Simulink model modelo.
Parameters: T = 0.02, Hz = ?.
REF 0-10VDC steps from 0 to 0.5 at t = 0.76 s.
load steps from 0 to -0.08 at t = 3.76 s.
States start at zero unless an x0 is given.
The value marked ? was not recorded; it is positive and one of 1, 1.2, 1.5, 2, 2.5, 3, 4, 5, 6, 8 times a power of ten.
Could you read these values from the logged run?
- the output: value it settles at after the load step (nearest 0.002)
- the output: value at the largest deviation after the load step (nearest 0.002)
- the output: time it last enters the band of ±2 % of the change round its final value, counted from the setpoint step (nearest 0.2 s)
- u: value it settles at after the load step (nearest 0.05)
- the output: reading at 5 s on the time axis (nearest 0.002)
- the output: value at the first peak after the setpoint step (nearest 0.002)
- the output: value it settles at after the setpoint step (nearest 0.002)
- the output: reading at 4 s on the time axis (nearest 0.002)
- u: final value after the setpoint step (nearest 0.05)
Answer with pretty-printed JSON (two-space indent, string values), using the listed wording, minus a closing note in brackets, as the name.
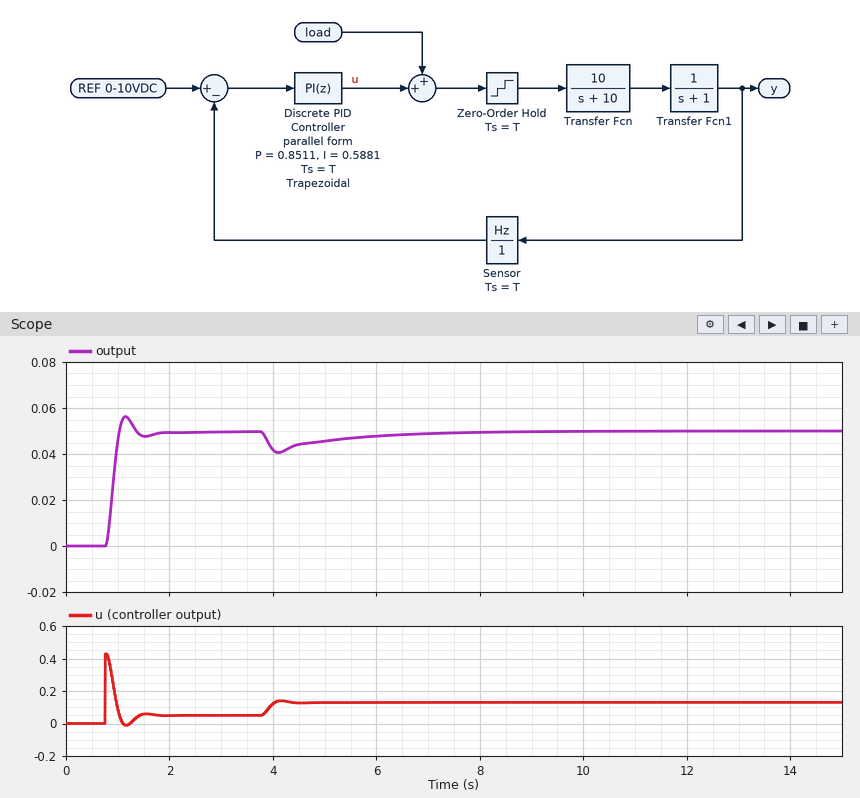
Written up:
{
  "the output: value it settles at after the load step": "0.050",
  "the output: value at the largest deviation after the load step": "0.040",
  "the output: time it last enters the band of ±2 % of the change round its final value, counted from the setpoint step": "1.0 s",
  "u: value it settles at after the load step": "0.15",
  "the output: reading at 5 s on the time axis": "0.046",
  "the output: value at the first peak after the setpoint step": "0.056",
  "the output: value it settles at after the setpoint step": "0.050",
  "the output: reading at 4 s on the time axis": "0.042",
  "u: final value after the setpoint step": "0.05"
}
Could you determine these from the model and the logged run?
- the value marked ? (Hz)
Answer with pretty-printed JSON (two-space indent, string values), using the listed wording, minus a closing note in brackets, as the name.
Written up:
{
  "the value marked ?": "10"
}
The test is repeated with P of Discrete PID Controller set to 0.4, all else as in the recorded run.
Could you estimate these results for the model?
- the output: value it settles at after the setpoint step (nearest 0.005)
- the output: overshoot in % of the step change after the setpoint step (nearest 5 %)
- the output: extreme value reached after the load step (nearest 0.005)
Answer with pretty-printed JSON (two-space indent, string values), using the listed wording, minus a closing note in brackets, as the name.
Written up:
{
  "the output: value it settles at after the setpoint step": "0.050",
  "the output: overshoot in % of the step change after the setpoint step": "10 %",
  "the output: extreme value reached after the load step": "0.035"
}
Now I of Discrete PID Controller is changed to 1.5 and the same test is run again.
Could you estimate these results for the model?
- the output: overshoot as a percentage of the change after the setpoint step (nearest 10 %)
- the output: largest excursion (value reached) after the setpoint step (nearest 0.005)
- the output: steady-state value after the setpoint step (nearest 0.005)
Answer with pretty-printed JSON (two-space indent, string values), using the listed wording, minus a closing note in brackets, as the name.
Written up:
{
  "the output: overshoot as a percentage of the change after the setpoint step": "30 %",
  "the output: largest excursion (value reached) after the setpoint step": "0.065",
  "the output: steady-state value after the setpoint step": "0.050"
}
